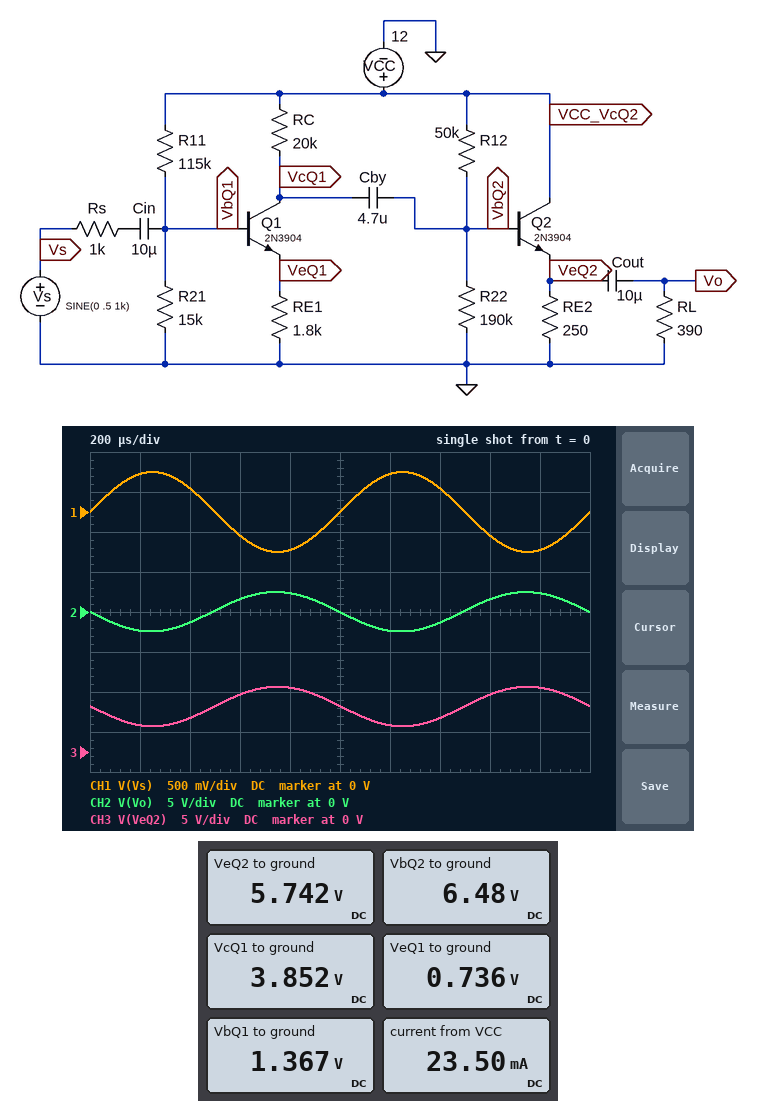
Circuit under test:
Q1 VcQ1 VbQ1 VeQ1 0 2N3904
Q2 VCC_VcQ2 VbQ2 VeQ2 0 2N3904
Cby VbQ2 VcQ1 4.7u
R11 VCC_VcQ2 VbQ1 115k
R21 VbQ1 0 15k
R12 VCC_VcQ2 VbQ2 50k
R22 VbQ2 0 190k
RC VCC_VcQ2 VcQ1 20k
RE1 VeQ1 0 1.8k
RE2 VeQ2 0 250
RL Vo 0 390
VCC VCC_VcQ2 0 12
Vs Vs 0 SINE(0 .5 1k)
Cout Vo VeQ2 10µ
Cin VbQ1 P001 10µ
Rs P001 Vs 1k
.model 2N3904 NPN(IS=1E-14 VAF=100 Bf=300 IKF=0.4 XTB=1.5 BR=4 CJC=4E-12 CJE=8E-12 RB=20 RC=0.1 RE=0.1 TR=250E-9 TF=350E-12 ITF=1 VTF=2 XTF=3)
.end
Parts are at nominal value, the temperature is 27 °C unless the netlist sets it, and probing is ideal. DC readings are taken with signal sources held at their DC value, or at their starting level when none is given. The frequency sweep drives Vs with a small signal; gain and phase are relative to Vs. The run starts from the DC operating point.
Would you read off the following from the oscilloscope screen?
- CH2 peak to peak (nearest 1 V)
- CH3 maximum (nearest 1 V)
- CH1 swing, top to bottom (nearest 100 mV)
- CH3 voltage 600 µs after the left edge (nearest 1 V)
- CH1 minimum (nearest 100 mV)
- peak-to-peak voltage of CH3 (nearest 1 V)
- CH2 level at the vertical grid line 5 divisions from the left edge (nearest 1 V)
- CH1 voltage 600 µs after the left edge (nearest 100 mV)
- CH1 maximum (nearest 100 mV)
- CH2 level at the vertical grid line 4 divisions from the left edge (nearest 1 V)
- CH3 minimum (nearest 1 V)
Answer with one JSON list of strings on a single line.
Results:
["5 V", "8 V", "1.0 V", "7 V", "-500 mV", "5 V", "0 V", "-300 mV", "500 mV", "2 V", "3 V"]
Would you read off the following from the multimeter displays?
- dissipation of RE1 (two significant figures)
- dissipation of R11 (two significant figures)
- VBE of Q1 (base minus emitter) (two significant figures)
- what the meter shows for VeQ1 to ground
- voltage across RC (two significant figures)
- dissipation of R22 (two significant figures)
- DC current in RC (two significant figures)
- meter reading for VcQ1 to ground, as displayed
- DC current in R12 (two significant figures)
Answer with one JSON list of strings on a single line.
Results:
["300 µW", "980 µW", "630 mV", "0.736 V", "8.1 V", "220 µW", "410 µA", "3.852 V", "110 µA"]
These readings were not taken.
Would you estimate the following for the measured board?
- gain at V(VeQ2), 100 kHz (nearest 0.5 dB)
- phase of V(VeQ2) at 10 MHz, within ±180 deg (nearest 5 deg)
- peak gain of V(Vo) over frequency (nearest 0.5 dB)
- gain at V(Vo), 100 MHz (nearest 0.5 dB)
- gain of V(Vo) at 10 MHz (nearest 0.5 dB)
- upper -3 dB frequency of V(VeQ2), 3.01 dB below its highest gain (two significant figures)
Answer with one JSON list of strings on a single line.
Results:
["14.0 dB", "75 deg", "14.0 dB", "-13.0 dB", "0 dB", "1.6 MHz"]
